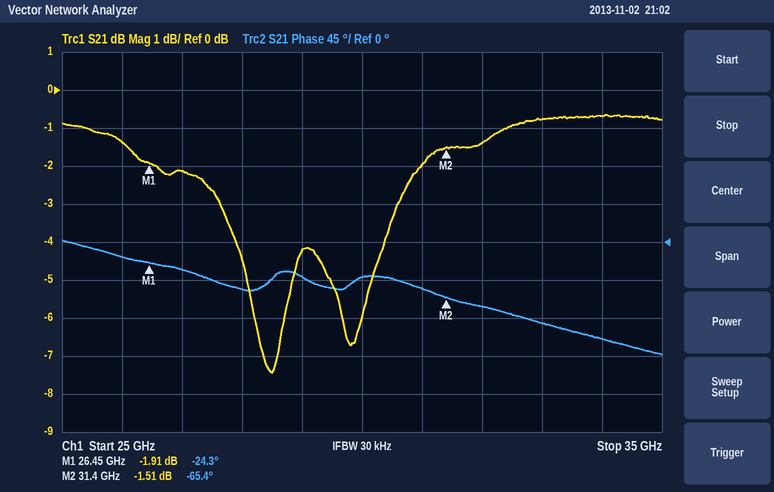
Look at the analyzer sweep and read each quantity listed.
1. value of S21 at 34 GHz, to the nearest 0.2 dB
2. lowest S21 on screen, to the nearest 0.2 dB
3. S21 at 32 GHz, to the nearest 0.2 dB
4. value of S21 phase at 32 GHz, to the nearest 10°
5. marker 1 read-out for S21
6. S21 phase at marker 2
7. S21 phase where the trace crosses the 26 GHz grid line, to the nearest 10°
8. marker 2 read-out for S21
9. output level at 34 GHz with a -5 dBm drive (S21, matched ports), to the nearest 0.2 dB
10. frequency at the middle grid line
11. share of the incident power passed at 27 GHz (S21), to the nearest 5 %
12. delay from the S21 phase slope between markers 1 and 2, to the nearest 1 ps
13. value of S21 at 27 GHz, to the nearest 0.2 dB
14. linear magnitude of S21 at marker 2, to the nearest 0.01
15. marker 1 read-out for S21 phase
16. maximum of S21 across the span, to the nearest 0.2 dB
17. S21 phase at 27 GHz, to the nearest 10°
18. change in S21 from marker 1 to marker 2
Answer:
-0.6 dB
-7.4 dB
-1.4 dB
-80°
-1.91 dB
-65.4°
-20°
-1.51 dB
-5.6 dBm
30 GHz
60 %
23 ps
-2.2 dB
0.84
-24.3°
-0.6 dB
-30°
0.40 dB
